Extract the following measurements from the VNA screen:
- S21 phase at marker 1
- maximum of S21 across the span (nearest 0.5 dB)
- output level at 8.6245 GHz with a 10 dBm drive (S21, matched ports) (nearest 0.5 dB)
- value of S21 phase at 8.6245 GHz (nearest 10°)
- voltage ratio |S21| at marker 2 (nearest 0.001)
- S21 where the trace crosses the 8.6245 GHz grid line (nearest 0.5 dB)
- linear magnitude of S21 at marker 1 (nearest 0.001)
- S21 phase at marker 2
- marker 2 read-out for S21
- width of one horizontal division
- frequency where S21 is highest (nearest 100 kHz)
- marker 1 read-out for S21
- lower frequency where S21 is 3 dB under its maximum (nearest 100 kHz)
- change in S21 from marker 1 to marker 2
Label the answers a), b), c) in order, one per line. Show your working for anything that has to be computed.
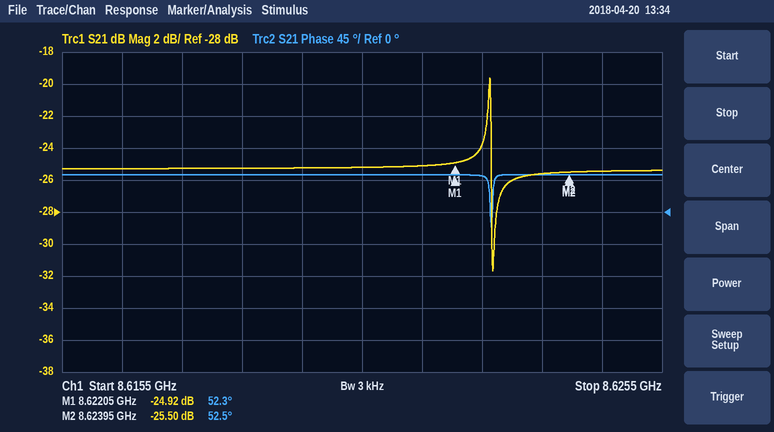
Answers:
a) 52.3°
b) -19.5 dB
c) 10 dBm + (-25.5 dB) = -15.5 dBm
d) 50°
e) 10^(-25.5/20) ≈ 0.053
f) -25.5 dB
g) 10^(-24.92/20) ≈ 0.057
h) 52.5°
i) -25.50 dB
j) 1 MHz
k) 8.6226 GHz
l) -24.92 dB
m) 8.6226 GHz
n) -25.5 − (-24.92) = -0.58 dB
